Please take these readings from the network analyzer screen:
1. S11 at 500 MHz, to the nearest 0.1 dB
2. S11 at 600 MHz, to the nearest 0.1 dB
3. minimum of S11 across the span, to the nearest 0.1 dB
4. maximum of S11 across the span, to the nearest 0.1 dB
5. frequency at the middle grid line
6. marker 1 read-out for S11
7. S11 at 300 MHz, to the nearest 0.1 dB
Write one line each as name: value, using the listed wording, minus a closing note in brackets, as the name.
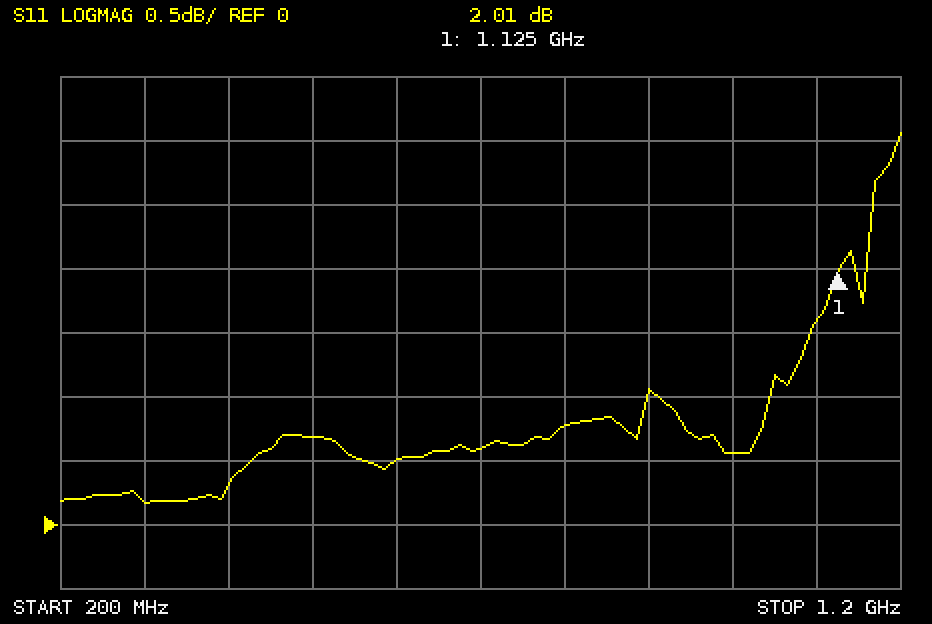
S11 at 500 MHz, to the nearest 0.1 dB: 0.7 dB
S11 at 600 MHz, to the nearest 0.1 dB: 0.5 dB
minimum of S11 across the span, to the nearest 0.1 dB: 0.2 dB
maximum of S11 across the span, to the nearest 0.1 dB: 3.1 dB
frequency at the middle grid line: 700 MHz
marker 1 read-out for S11: 2.01 dB
S11 at 300 MHz, to the nearest 0.1 dB: 0.2 dB
